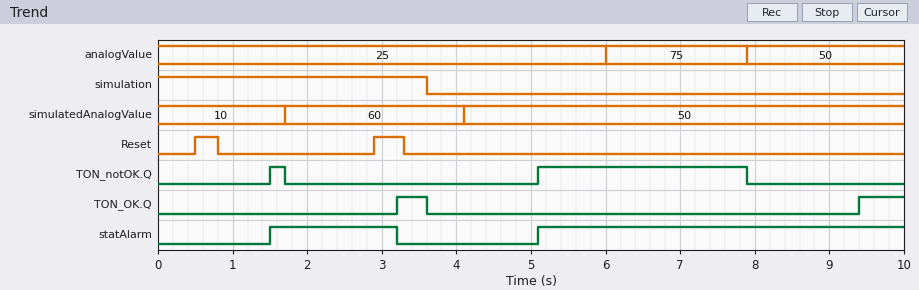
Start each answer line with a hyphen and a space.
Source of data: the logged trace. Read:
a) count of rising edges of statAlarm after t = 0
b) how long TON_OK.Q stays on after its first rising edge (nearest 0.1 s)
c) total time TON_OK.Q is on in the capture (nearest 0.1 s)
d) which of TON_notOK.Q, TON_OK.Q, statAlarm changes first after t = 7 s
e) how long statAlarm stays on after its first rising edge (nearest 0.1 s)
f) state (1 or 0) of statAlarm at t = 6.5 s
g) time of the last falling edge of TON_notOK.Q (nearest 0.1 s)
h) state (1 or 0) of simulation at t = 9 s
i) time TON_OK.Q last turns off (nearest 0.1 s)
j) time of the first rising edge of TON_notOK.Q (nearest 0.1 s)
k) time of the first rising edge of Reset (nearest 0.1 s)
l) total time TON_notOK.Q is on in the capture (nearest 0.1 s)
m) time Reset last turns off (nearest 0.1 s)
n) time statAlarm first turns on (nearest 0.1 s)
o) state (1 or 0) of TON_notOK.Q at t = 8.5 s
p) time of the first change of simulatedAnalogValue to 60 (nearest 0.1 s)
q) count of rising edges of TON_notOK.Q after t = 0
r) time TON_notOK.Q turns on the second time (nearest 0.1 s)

- 2
- 0.4 s
- 1.0 s
- TON_notOK.Q
- 1.7 s
- 1
- 7.9 s
- 0
- 3.6 s
- 1.5 s
- 0.5 s
- 3.0 s
- 3.3 s
- 1.5 s
- 0
- 1.7 s
- 2
- 5.1 s
